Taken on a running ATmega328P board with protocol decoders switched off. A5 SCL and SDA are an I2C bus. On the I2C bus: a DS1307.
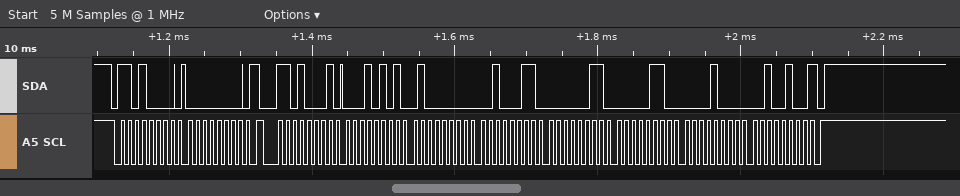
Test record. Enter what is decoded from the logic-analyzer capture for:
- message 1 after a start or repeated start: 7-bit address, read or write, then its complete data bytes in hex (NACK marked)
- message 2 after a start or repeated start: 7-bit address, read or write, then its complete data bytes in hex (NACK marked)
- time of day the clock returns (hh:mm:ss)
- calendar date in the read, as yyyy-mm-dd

0x68 write: 00
0x68 read: 15 40 23 03 06 08 24 NACK
23:40:15
2024-08-06
